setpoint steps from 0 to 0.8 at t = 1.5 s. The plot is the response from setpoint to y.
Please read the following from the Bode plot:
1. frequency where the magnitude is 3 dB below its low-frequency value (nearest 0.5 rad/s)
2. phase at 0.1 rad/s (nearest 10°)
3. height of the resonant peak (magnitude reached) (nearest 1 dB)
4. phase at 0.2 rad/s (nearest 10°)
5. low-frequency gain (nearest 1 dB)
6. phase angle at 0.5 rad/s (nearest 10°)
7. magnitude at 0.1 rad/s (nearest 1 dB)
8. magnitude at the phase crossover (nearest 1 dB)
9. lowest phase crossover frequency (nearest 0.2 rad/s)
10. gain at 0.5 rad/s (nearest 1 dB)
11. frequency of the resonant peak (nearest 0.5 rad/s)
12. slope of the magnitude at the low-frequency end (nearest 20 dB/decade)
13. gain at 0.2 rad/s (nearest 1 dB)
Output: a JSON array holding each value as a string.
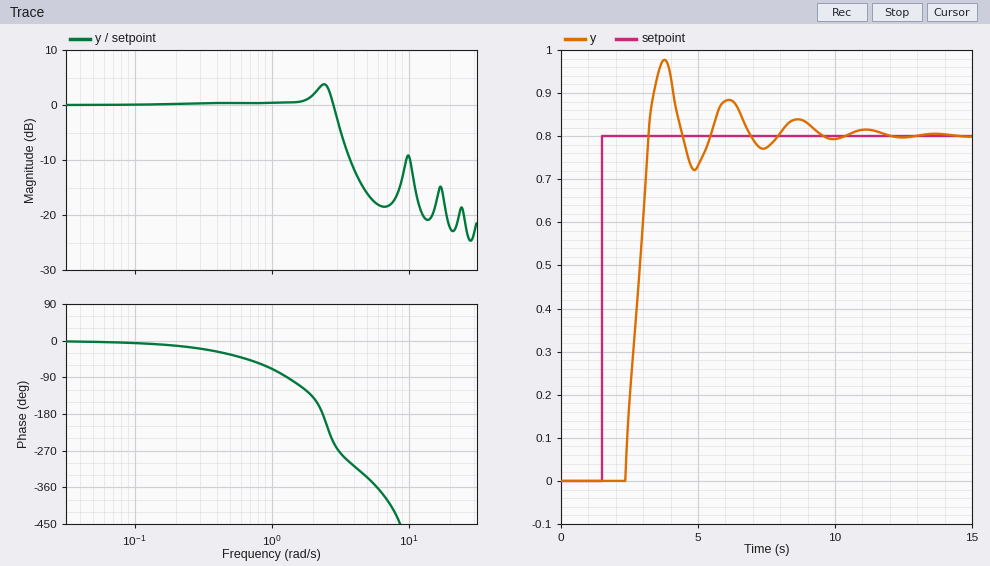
["3.0 rad/s", "-10°", "4 dB", "-10°", "0 dB", "-30°", "0 dB", "4 dB", "2.4 rad/s", "0 dB", "2.5 rad/s", "0 dB/decade", "0 dB"]
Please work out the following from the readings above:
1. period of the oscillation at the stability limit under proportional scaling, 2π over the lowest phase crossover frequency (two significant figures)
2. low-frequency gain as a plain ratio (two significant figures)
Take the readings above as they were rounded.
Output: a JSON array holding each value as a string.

["2.6 s", "1.0"]
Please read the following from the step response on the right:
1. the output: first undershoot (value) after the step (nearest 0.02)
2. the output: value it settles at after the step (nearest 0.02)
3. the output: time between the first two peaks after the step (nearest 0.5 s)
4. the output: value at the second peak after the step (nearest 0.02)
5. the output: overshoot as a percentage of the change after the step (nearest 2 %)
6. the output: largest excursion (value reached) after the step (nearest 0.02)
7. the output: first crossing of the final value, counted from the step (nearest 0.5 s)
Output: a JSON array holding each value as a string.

["0.72", "0.80", "2.5 s", "0.88", "22 %", "0.98", "1.5 s"]
